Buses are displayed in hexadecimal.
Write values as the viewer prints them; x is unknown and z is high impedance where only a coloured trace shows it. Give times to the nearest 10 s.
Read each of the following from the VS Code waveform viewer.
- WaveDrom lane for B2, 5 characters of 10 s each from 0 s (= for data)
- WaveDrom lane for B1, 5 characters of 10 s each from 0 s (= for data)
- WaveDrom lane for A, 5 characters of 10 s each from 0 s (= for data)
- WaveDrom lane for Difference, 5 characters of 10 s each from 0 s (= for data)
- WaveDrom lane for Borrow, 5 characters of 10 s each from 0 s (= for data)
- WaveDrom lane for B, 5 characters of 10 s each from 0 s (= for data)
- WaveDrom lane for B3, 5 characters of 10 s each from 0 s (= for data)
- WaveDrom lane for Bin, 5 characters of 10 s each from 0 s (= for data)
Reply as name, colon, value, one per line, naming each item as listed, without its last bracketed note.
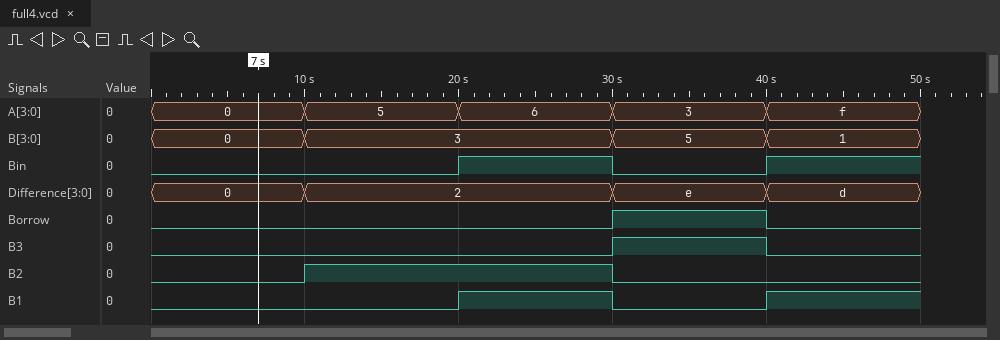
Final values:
WaveDrom lane for B2, 5 characters of 10 s each from 0 s: {name: 'B2', wave: '01.0.'}
WaveDrom lane for B1, 5 characters of 10 s each from 0 s: {name: 'B1', wave: '0.101'}
WaveDrom lane for A, 5 characters of 10 s each from 0 s: {name: 'A', wave: '=====', data: '0 5 6 3 f'}
WaveDrom lane for Difference, 5 characters of 10 s each from 0 s: {name: 'Difference', wave: '==.==', data: '0 2 e d'}
WaveDrom lane for Borrow, 5 characters of 10 s each from 0 s: {name: 'Borrow', wave: '0..10'}
WaveDrom lane for B, 5 characters of 10 s each from 0 s: {name: 'B', wave: '==.==', data: '0 3 5 1'}
WaveDrom lane for B3, 5 characters of 10 s each from 0 s: {name: 'B3', wave: '0..10'}
WaveDrom lane for Bin, 5 characters of 10 s each from 0 s: {name: 'Bin', wave: '0.101'}
